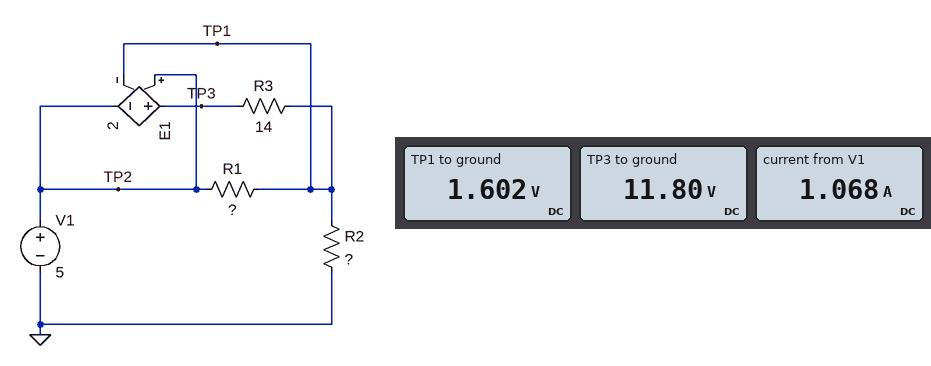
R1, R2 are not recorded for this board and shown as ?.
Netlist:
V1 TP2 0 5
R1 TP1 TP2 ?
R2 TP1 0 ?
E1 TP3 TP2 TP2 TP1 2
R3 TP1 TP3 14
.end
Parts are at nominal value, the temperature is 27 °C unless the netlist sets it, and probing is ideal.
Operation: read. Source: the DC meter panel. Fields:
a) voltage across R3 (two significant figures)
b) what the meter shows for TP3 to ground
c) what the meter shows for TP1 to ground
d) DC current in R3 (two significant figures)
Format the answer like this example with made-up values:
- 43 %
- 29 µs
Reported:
- 10 V
- 11.80 V
- 1.602 V
- 730 mA
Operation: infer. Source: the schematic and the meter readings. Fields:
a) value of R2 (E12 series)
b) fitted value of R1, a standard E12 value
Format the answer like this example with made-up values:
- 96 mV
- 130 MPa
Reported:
- 1.5 Ω
- 10 Ω
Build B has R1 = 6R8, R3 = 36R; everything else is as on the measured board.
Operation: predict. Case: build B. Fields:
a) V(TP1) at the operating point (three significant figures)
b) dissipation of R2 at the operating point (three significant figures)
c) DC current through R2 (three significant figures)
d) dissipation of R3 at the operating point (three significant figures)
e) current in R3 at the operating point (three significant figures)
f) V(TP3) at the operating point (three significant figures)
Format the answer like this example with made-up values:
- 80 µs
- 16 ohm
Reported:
- 1.28 V
- 1.10 W
- 856 mA
- 3.45 W
- 310 mA
- 12.4 V
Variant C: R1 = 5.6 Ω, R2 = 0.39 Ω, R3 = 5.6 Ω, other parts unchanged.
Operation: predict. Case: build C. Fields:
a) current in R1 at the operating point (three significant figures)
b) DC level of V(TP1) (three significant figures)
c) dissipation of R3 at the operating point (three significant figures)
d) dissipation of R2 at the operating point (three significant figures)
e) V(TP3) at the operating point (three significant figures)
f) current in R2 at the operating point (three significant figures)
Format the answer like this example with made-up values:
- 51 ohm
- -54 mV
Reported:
- 698 mA
- 1.09 V
- 24.6 W
- 3.04 W
- 12.8 V
- 2.79 A
